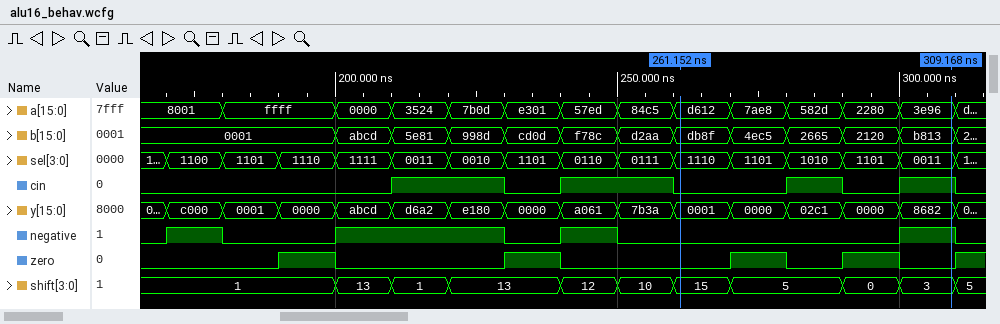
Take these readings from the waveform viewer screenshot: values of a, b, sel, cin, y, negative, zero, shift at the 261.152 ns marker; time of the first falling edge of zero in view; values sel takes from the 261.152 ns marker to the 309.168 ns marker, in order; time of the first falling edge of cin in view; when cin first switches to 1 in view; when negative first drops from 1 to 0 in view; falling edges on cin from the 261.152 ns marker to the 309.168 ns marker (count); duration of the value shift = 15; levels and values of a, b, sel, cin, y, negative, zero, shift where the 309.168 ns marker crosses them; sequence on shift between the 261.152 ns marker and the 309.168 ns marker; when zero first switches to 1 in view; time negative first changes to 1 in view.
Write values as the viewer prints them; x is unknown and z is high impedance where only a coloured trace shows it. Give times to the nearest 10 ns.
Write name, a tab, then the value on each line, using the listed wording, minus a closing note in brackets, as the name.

values of a, b, sel, cin, y, negative, zero, shift at the 261.152 ns marker	a=d612, b=db8f, sel=1110, cin=0, y=0001, negative=0, zero=0, shift=15
time of the first falling edge of zero in view	200 ns
values sel takes from the 261.152 ns marker to the 309.168 ns marker, in order	1110, 1101, 1010, 1101, 0011
time of the first falling edge of cin in view	230 ns
when cin first switches to 1 in view	210 ns
when negative first drops from 1 to 0 in view	180 ns
falling edges on cin from the 261.152 ns marker to the 309.168 ns marker	1
duration of the value shift = 15	10 ns
levels and values of a, b, sel, cin, y, negative, zero, shift where the 309.168 ns marker crosses them	a=3e96, b=b813, sel=0011, cin=1, y=8682, negative=1, zero=0, shift=3
sequence on shift between the 261.152 ns marker and the 309.168 ns marker	15, 5, 0, 3
when zero first switches to 1 in view	190 ns
time negative first changes to 1 in view	170 ns
